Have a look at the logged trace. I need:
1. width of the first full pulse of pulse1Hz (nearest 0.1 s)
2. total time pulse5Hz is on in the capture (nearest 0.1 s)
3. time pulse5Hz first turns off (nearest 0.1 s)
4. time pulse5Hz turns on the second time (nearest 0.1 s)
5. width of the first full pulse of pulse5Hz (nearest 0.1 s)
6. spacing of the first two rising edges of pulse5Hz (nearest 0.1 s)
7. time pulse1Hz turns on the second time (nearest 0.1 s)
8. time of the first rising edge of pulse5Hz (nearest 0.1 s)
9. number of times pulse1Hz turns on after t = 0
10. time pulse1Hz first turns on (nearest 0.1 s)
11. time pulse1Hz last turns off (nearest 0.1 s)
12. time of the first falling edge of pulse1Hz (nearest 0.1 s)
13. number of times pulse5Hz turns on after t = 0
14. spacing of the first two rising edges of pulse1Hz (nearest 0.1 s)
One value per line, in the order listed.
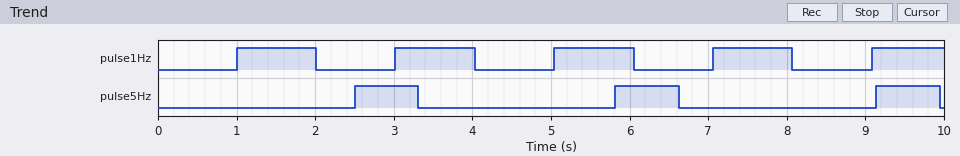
1.0 s
2.4 s
3.3 s
5.8 s
0.8 s
3.3 s
3.0 s
2.5 s
5
1.0 s
8.1 s
2.0 s
3
2.0 s
